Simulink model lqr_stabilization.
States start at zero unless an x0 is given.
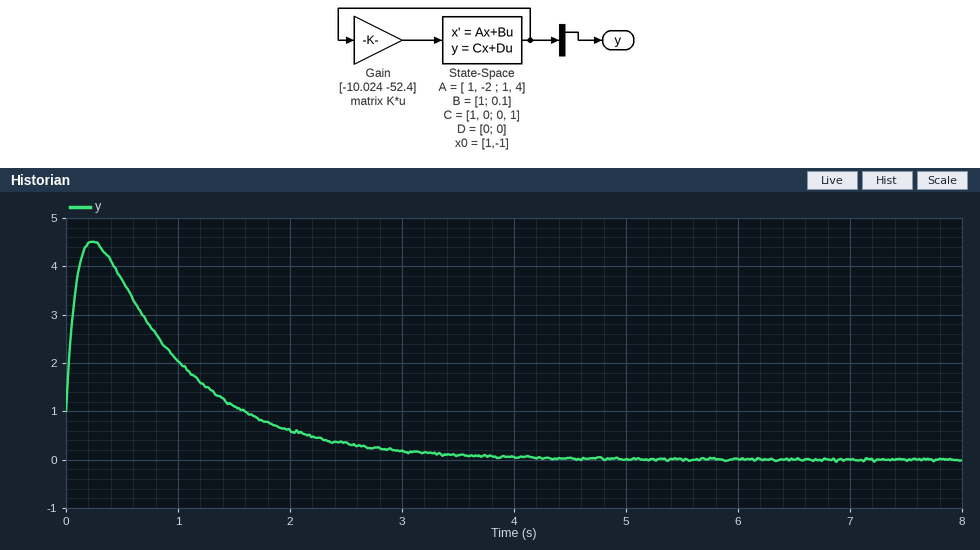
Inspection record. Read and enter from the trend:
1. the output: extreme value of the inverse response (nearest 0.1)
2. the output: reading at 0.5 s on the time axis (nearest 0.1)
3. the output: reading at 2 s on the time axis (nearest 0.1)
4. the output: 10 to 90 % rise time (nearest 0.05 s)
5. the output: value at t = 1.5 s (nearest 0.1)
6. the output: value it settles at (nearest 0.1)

4.5
3.7
0.6
1.80 s
1.1
0.0
